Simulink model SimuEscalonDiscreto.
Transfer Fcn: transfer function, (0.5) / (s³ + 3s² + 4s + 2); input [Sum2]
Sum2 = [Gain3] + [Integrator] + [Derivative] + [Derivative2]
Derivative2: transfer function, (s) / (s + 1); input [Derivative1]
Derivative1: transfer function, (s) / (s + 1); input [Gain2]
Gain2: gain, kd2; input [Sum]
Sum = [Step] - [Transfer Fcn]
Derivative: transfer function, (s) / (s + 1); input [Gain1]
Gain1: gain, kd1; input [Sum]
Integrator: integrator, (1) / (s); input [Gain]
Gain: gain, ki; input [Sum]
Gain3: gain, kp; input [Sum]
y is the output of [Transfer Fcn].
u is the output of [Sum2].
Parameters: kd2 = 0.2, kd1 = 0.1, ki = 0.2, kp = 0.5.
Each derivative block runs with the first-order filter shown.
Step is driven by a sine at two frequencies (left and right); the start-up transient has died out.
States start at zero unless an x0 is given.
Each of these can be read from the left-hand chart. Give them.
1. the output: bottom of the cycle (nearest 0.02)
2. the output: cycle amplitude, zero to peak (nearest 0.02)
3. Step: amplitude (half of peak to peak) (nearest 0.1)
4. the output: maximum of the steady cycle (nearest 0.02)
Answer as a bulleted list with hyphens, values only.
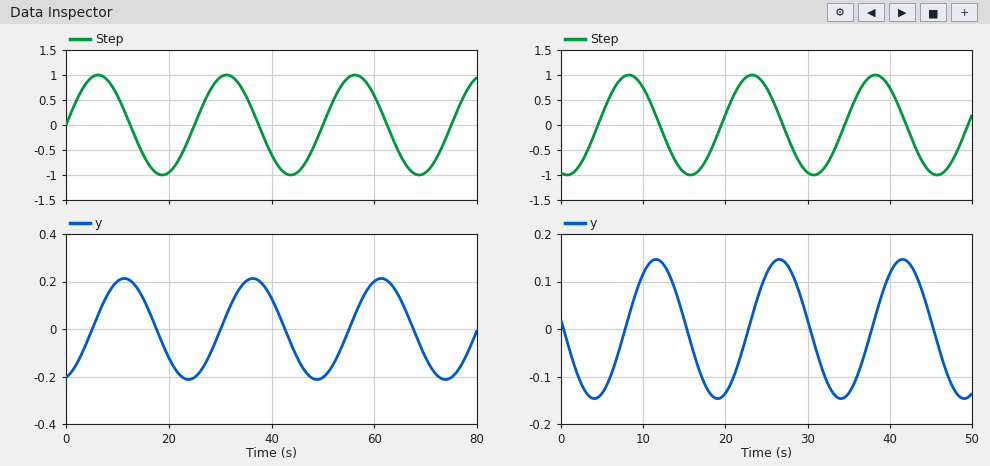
- -0.22
- 0.22
- 1.0
- 0.22
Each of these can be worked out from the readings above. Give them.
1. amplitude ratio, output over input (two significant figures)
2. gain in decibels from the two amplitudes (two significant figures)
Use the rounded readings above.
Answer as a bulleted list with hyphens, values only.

- 0.22
- -13 dB
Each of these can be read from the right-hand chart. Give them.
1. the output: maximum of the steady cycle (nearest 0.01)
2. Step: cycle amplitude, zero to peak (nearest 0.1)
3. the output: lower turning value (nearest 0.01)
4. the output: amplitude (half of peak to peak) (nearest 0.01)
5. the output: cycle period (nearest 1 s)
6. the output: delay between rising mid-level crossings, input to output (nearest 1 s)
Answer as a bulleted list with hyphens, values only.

- 0.15
- 1.0
- -0.15
- 0.15
- 15 s
- 3 s
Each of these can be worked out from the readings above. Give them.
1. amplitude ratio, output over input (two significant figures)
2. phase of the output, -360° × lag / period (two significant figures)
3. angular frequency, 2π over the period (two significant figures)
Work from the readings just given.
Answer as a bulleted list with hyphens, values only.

- 0.15
- -72°
- 0.42 rad/s
